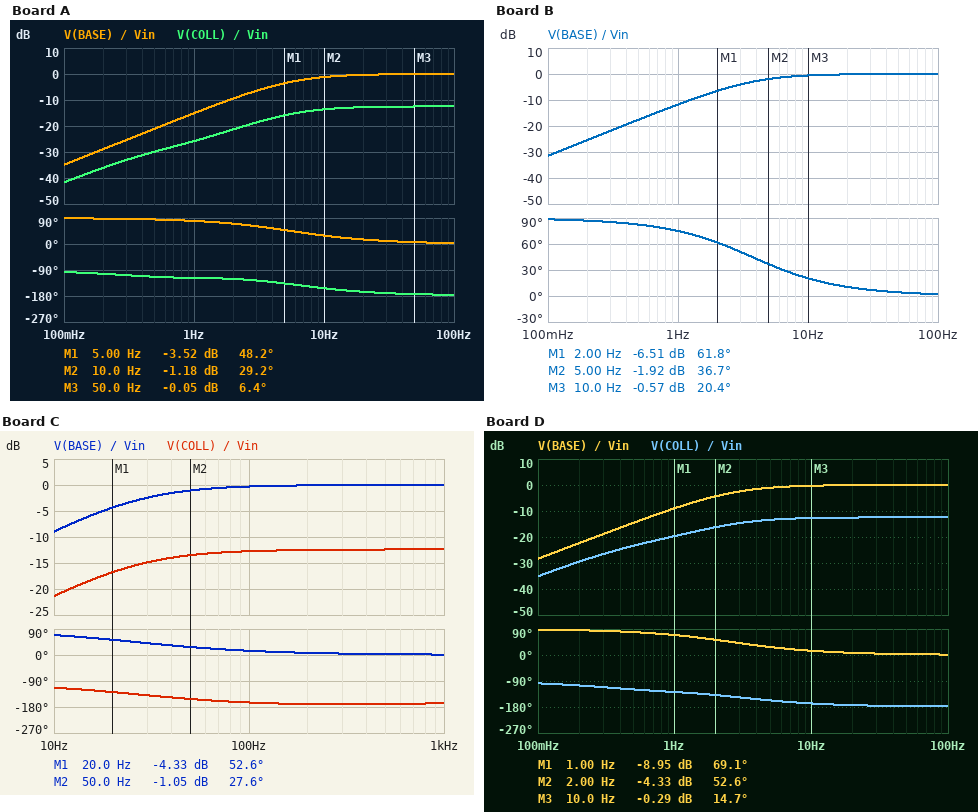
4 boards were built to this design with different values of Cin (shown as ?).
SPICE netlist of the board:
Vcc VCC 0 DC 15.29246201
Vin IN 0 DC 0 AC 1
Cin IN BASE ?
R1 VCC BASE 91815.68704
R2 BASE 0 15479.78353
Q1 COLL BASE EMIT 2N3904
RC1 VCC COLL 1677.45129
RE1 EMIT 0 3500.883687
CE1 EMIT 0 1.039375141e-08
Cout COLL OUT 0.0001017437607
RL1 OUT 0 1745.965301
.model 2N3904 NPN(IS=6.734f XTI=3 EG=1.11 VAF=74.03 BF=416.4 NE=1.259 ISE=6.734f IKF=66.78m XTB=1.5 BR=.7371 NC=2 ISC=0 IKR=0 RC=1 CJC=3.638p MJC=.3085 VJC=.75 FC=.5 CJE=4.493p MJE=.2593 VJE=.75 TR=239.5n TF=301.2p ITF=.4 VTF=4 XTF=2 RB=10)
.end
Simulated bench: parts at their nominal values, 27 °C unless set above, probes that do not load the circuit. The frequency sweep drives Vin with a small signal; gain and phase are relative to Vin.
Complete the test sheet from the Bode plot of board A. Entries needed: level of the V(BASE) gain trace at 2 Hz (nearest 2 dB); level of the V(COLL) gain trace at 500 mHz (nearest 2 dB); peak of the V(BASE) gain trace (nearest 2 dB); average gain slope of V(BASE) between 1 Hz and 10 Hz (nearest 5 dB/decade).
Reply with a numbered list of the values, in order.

1. -10 dB
2. -30 dB
3. 0 dB
4. 15 dB/decade
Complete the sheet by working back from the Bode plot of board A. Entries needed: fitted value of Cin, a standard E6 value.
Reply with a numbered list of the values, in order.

1. 2.2 µF
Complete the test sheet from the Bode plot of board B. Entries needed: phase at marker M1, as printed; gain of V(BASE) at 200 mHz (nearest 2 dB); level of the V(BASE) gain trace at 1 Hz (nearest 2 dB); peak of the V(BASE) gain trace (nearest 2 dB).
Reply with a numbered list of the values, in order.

1. 61.8 deg
2. -26 dB
3. -12 dB
4. 0 dB
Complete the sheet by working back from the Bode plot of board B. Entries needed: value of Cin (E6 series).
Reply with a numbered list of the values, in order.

1. 3.3 µF
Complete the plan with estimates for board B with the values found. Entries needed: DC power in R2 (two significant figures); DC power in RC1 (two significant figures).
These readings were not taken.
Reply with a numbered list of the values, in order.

1. 300 µW
2. 310 µW
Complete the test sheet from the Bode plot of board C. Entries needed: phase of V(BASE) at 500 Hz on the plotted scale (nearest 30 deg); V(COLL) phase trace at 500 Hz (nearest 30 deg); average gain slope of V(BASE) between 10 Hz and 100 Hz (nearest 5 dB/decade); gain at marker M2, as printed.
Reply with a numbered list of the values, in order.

1. 0 deg
2. -180 deg
3. 10 dB/decade
4. -1.05 dB
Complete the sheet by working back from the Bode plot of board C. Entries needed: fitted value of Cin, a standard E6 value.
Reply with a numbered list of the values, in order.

1. 470 nF
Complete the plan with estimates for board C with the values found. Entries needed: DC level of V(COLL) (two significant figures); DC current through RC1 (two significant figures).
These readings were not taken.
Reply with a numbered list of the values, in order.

1. 15 V
2. 430 µA
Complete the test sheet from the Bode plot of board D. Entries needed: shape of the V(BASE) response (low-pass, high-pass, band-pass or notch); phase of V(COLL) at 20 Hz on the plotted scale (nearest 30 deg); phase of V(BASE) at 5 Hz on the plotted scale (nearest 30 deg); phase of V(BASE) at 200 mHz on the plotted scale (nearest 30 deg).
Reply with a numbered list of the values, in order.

1. high-pass
2. -180 deg
3. 30 deg
4. 90 deg
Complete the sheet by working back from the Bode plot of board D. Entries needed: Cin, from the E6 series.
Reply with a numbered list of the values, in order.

1. 4.7 µF
